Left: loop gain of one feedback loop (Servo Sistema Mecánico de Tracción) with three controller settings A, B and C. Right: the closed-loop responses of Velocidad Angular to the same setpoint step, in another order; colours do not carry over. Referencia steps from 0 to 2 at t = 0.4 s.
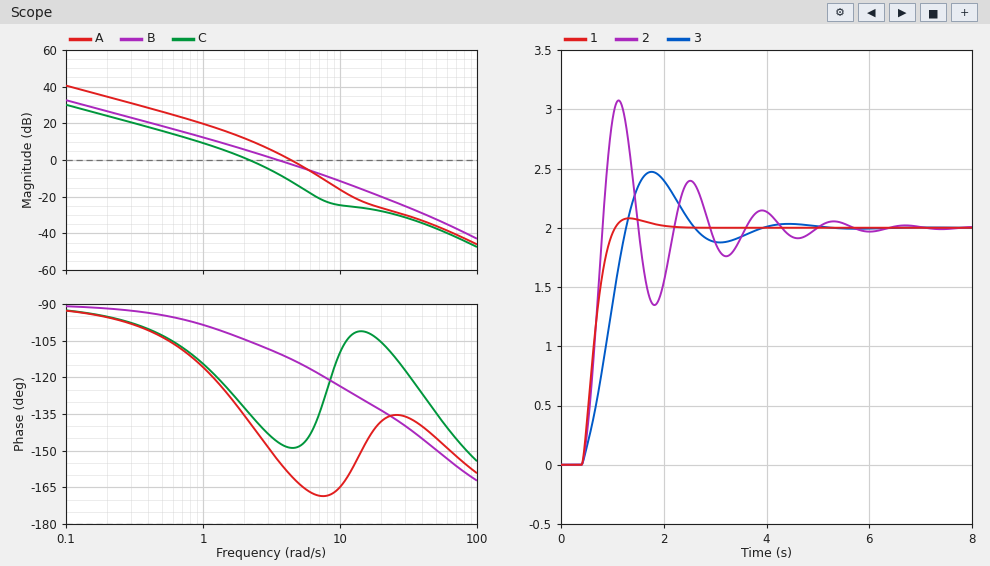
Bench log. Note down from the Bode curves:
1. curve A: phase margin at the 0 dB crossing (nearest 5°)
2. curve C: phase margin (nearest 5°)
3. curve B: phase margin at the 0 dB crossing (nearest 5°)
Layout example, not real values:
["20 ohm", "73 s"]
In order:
["20°", "45°", "70°"]
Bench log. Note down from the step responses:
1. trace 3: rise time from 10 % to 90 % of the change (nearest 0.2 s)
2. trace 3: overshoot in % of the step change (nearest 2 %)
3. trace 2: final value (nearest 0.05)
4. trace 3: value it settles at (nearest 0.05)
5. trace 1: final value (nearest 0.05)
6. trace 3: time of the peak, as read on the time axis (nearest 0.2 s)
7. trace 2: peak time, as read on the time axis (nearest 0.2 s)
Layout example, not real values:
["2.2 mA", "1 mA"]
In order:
["0.6 s", "24 %", "2.00", "2.00", "2.00", "1.8 s", "1.2 s"]
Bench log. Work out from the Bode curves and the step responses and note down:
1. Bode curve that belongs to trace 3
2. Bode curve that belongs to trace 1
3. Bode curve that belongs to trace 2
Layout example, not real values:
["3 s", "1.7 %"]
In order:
["C", "B", "A"]
